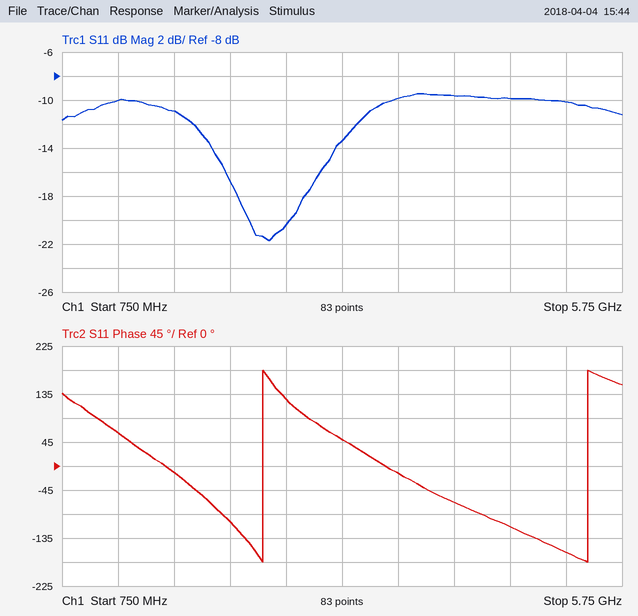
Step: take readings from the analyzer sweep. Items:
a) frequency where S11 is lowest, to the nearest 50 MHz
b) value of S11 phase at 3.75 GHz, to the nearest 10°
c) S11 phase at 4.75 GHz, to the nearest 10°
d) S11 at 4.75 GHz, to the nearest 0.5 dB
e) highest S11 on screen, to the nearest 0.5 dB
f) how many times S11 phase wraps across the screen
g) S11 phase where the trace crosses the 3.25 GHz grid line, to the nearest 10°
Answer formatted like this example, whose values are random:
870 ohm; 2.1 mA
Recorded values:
2.60 GHz; -10°; -110°; -10.0 dB; -9.5 dB; 2; 50°
